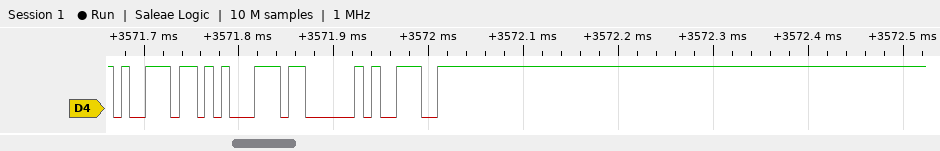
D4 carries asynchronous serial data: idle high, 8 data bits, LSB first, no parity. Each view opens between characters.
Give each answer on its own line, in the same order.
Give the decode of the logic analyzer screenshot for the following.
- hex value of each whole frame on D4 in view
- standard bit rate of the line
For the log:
B9, C5, 03, 39
115200 baud
